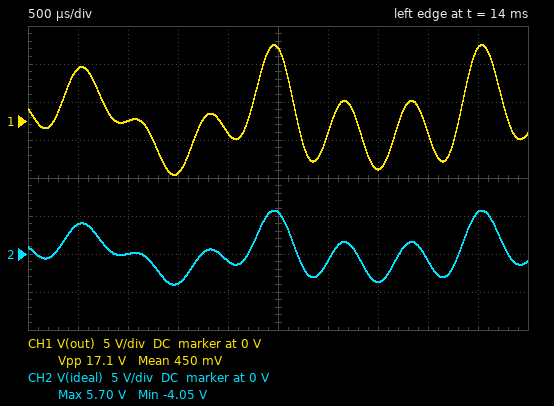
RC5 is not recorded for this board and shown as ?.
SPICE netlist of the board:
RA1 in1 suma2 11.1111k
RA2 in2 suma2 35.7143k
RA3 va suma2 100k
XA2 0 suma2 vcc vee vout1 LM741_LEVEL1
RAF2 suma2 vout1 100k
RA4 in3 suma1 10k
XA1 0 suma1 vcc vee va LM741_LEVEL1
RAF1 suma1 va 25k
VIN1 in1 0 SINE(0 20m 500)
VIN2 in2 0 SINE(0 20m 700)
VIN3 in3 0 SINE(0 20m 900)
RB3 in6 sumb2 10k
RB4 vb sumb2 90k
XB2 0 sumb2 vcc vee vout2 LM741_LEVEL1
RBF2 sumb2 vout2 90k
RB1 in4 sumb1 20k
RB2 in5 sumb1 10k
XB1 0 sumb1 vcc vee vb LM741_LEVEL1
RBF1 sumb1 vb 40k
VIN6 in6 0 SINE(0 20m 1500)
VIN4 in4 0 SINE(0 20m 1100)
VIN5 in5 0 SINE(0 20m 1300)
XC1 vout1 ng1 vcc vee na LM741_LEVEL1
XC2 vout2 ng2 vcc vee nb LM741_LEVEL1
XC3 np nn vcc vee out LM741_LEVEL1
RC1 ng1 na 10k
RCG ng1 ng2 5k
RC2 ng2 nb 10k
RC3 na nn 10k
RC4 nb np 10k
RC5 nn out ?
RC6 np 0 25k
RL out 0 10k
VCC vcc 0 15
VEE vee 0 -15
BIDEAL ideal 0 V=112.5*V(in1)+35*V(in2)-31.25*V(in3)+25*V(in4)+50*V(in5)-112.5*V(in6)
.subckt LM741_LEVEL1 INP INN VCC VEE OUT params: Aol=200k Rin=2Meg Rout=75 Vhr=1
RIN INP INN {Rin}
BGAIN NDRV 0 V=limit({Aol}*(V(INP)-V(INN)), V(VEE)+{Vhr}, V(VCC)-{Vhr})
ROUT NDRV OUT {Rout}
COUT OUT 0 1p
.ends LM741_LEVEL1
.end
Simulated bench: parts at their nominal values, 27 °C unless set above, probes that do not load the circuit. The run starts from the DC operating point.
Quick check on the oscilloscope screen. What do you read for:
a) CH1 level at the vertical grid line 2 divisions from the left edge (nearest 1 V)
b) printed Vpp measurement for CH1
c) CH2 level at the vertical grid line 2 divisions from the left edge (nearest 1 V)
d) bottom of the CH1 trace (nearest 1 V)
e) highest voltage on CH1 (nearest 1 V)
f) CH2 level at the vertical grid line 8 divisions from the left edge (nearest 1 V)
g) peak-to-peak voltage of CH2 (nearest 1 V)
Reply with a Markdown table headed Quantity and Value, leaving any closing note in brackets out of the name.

| Quantity | Value |
|---|---|
| CH1 level at the vertical grid line 2 divisions from the left edge | 0 V |
| printed Vpp measurement for CH1 | 17.1 V |
| CH2 level at the vertical grid line 2 divisions from the left edge | 0 V |
| bottom of the CH1 trace | -7 V |
| highest voltage on CH1 | 10 V |
| CH2 level at the vertical grid line 8 divisions from the left edge | -1 V |
| peak-to-peak voltage of CH2 | 10 V |
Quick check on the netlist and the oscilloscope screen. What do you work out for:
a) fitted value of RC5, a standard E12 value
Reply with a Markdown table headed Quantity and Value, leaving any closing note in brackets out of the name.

| Quantity | Value |
|---|---|
| fitted value of RC5, a standard E12 value | 47 kΩ |
